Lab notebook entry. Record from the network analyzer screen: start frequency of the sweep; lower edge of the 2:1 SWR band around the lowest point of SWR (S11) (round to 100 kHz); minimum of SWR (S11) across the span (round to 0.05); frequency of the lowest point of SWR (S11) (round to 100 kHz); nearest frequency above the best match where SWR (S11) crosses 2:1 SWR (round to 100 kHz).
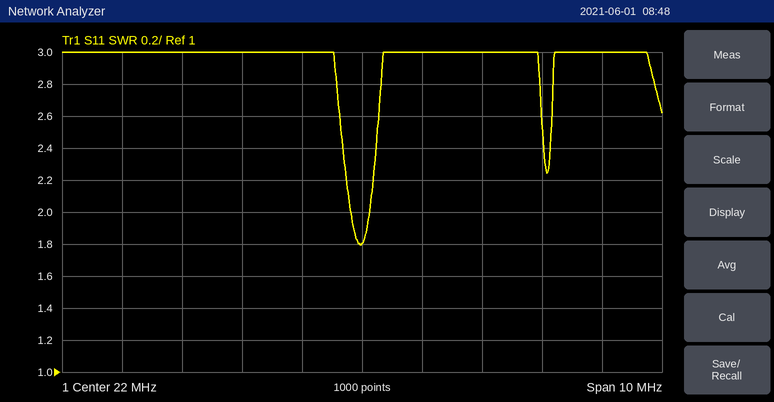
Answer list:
17 MHz
21.8 MHz
1.80
22.0 MHz
22.1 MHz
